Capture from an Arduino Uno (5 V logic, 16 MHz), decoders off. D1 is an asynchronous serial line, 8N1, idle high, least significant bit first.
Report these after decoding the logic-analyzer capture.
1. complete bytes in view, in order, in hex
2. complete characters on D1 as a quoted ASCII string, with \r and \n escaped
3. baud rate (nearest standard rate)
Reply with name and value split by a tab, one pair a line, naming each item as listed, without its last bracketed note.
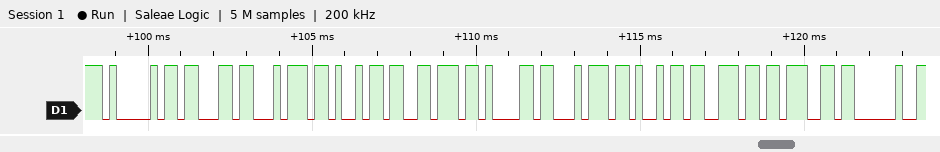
complete bytes in view, in order, in hex	0x41 0x63 0x74 0x69 0x76 0x61 0x74 0x69 0x6E 0x67 0x20
complete characters on D1 as a quoted ASCII string, with \r and \n escaped	"Activating "
baud rate	4800 baud
